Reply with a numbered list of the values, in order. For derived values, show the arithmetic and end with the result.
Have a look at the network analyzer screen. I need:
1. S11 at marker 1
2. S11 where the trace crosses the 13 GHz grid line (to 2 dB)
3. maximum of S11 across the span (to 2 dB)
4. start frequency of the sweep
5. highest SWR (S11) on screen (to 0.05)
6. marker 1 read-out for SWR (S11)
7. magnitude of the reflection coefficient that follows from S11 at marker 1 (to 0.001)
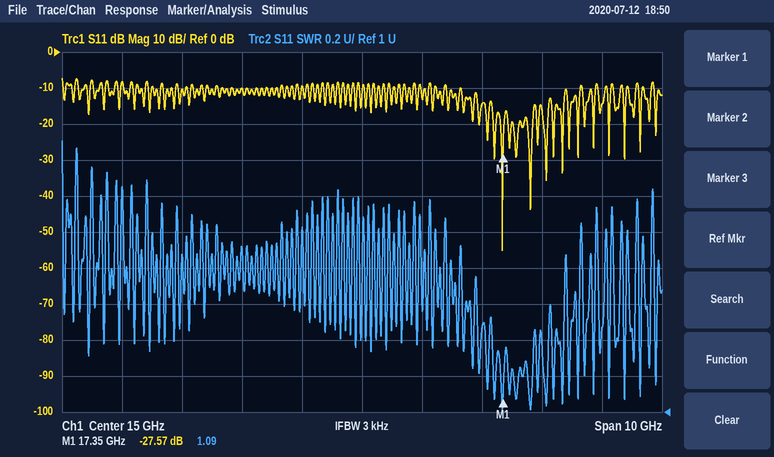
1. -27.57 dB
2. -10 dB
3. -8 dB
4. 10 GHz
5. 2.50
6. 1.09
7. 10^(-27.57/20) ≈ 0.042
